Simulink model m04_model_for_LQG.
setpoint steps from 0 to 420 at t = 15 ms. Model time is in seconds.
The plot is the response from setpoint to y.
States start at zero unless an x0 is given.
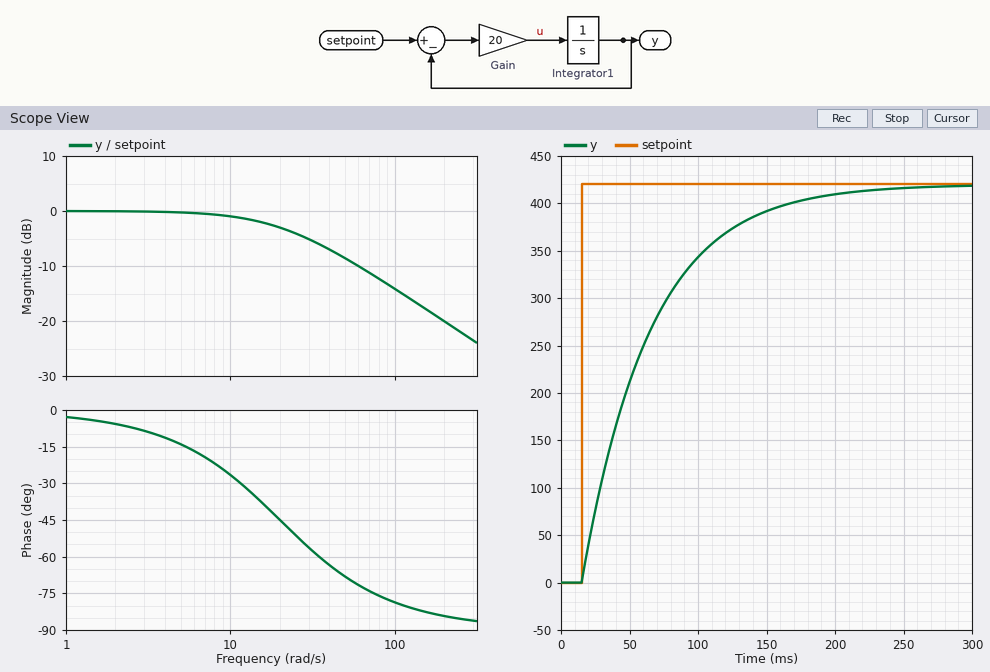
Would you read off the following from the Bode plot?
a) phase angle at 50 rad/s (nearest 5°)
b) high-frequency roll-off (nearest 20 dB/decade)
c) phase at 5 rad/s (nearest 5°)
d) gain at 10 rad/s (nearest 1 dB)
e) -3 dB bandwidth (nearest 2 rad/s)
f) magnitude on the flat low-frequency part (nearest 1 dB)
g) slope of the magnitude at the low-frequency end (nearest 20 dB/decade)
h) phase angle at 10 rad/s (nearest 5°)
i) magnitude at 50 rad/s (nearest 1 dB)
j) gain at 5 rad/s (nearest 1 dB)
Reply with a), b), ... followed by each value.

a) -70°
b) -20 dB/decade
c) -15°
d) -1 dB
e) 20 rad/s
f) 0 dB
g) 0 dB/decade
h) -25°
i) -9 dB
j) 0 dB
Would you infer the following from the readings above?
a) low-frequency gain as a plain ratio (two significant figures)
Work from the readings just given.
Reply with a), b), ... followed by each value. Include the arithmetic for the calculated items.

a) 10^(0 / 20) = 1.0
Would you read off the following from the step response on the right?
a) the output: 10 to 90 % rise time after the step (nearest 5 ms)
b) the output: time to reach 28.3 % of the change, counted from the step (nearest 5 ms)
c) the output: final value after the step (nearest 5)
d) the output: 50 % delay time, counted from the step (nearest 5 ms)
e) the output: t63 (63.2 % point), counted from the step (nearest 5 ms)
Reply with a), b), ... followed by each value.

a) 110 ms
b) 15 ms
c) 420
d) 35 ms
e) 50 ms
